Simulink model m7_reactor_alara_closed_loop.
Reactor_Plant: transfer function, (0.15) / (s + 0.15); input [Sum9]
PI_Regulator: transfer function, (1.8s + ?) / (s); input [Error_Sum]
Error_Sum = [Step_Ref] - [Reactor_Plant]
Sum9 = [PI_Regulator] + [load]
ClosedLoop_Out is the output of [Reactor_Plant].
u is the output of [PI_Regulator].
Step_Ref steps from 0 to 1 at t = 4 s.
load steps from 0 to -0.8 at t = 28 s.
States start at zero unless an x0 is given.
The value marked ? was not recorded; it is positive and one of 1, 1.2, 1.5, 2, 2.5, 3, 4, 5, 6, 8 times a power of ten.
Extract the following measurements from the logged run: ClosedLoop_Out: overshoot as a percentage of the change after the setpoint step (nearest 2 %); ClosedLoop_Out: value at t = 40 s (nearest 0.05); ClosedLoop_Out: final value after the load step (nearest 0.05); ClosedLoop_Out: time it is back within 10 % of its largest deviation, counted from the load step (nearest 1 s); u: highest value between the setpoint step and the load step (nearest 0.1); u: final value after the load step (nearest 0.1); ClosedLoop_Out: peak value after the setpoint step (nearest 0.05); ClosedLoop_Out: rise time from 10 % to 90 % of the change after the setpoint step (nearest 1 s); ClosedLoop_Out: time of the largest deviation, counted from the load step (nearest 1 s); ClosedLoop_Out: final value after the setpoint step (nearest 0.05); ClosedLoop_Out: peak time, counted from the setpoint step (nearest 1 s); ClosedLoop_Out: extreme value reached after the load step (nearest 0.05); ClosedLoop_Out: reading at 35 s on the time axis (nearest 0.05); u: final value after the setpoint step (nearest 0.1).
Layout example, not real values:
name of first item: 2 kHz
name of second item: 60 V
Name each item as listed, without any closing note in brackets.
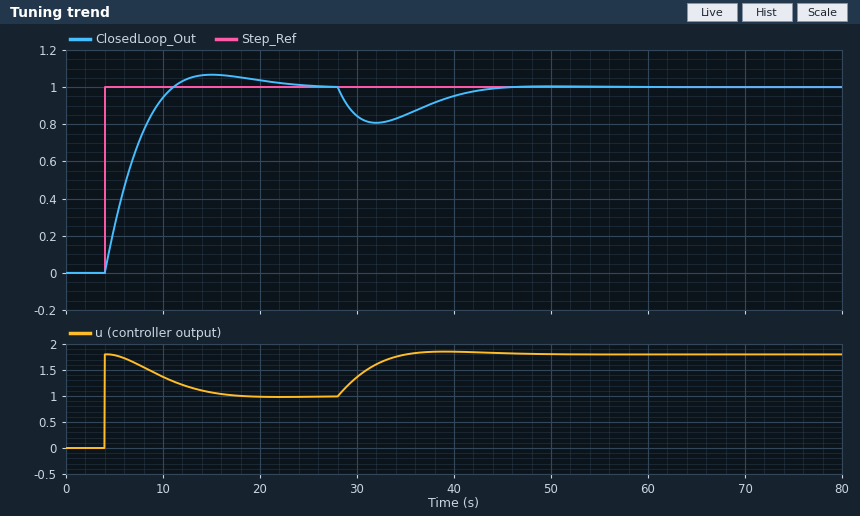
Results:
ClosedLoop_Out: overshoot as a percentage of the change after the setpoint step: 6 %
ClosedLoop_Out: value at t = 40 s: 0.95
ClosedLoop_Out: final value after the load step: 1.00
ClosedLoop_Out: time it is back within 10 % of its largest deviation, counted from the load step: 14 s
u: highest value between the setpoint step and the load step: 1.8
u: final value after the load step: 1.8
ClosedLoop_Out: peak value after the setpoint step: 1.05
ClosedLoop_Out: rise time from 10 % to 90 % of the change after the setpoint step: 5 s
ClosedLoop_Out: time of the largest deviation, counted from the load step: 4 s
ClosedLoop_Out: final value after the setpoint step: 1.00
ClosedLoop_Out: peak time, counted from the setpoint step: 11 s
ClosedLoop_Out: extreme value reached after the load step: 0.80
ClosedLoop_Out: reading at 35 s on the time axis: 0.85
u: final value after the setpoint step: 1.0
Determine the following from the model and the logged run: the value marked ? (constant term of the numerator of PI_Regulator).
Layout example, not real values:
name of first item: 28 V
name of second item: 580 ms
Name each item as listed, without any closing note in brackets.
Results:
the value marked ?: 0.5
